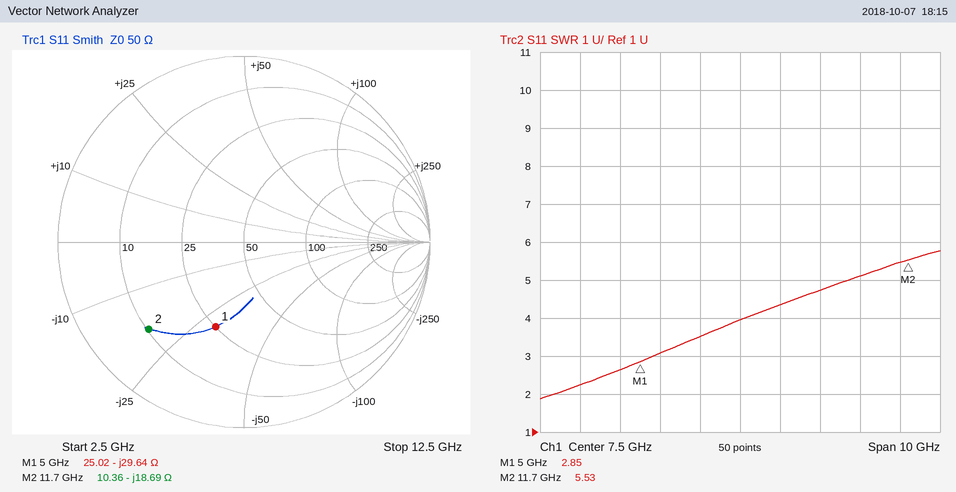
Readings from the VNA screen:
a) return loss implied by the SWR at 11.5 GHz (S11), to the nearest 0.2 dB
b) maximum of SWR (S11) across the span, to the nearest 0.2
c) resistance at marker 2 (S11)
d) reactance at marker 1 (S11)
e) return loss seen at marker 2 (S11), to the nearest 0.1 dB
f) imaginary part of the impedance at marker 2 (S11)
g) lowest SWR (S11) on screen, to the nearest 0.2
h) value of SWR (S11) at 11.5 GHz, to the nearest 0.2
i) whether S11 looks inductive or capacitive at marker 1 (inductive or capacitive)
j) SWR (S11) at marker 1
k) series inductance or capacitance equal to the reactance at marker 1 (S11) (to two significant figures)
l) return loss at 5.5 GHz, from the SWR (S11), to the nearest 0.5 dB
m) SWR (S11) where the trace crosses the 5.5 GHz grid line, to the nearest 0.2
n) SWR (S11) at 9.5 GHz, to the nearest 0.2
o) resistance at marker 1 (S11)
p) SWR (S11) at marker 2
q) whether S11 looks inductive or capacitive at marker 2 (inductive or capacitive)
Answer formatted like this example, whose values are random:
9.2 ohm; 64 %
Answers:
3.2 dB; 5.8; 10.36 Ω; -29.64 Ω; 3.2 dB; -18.69 Ω; 1.8; 5.4; capacitive; 2.85; 1.1 pF; 6.0 dB; 3.0; 4.8; 25.02 Ω; 5.53; capacitive
